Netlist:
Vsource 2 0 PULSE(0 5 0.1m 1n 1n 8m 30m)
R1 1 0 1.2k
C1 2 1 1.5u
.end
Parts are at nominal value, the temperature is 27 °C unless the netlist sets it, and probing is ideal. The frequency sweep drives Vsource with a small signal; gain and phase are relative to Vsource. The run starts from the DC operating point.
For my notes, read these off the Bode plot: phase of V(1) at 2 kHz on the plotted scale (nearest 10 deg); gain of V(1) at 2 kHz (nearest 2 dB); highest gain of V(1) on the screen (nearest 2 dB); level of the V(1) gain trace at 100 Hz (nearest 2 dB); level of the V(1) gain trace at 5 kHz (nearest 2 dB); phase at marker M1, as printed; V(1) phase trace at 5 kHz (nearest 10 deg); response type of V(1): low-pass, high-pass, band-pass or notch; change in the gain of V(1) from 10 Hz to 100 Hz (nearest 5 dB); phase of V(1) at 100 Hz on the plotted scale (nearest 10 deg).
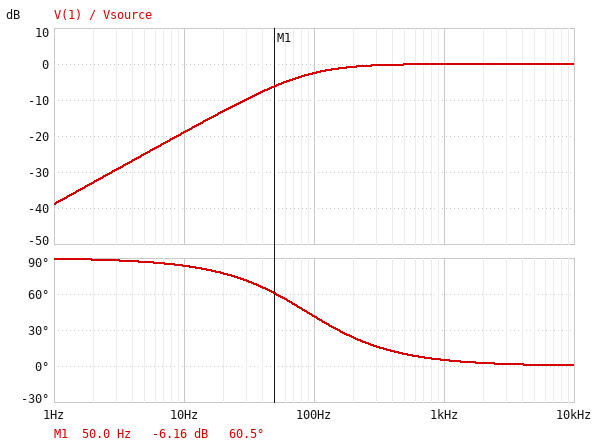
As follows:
0 deg
0 dB
0 dB
-2 dB
0 dB
60.5 deg
0 deg
high-pass
15 dB
40 deg
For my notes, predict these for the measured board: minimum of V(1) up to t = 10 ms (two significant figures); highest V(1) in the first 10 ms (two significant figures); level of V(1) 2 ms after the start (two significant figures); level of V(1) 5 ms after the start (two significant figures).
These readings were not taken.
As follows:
-4.9 V
5.0 V
1.7 V
330 mV
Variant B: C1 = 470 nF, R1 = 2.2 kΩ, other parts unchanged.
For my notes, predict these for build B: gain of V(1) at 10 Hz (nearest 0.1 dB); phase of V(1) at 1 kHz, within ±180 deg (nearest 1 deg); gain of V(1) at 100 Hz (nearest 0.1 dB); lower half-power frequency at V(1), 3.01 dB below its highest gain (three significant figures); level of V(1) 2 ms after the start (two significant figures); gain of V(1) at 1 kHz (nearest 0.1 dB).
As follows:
-23.8 dB
9 deg
-5.3 dB
154 Hz
800 mV
-0.1 dB
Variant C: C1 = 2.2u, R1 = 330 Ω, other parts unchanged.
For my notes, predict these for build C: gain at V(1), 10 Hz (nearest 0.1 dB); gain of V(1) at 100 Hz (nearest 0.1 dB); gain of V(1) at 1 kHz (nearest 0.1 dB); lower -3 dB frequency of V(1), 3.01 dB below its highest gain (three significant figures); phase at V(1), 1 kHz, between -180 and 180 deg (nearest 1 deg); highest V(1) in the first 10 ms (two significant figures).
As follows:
-26.8 dB
-7.6 dB
-0.2 dB
219 Hz
12 deg
5.0 V
